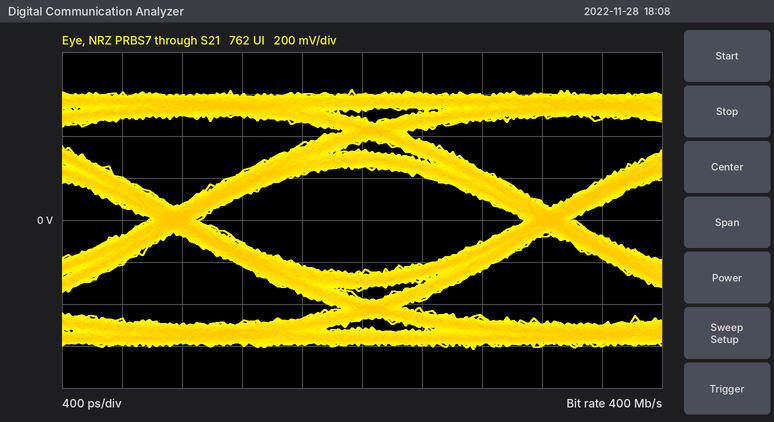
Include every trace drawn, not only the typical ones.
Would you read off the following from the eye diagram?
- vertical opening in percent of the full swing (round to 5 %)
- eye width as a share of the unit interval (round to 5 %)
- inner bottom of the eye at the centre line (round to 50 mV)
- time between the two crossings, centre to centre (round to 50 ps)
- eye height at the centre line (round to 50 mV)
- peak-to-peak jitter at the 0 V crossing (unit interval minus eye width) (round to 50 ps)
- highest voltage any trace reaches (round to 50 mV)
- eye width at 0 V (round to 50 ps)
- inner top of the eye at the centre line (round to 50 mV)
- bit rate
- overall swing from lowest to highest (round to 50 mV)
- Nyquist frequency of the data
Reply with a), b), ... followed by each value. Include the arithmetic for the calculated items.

a) 500 mV / 1.25 V ≈ 40 %
b) 2.15 ns / 2.50 ns ≈ 86.0 %, so 85 % to the nearest 5 %
c) -250 mV
d) 2.50 ns
e) 500 mV
f) 350 ps
g) 600 mV
h) 2.15 ns
i) 250 mV
j) 400 Mb/s
k) 1.25 V
l) 200 MHz
